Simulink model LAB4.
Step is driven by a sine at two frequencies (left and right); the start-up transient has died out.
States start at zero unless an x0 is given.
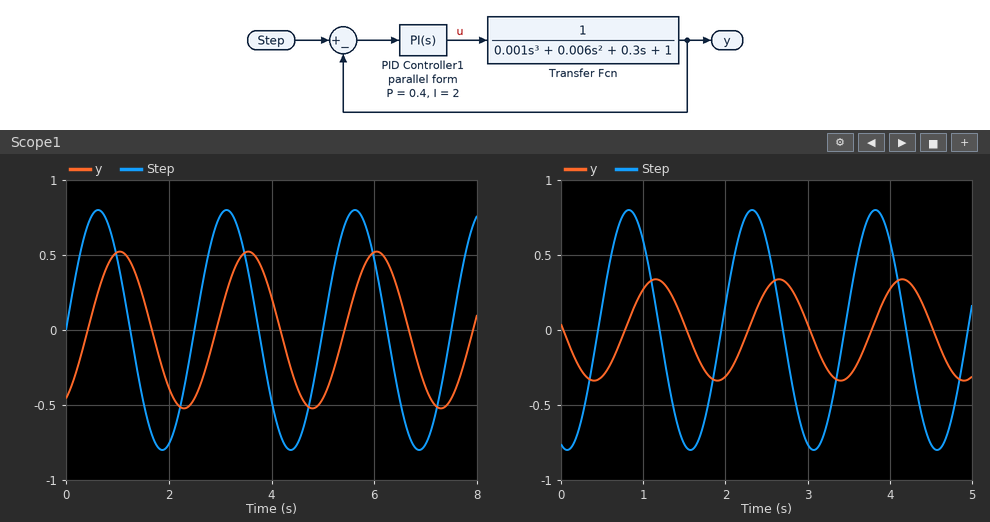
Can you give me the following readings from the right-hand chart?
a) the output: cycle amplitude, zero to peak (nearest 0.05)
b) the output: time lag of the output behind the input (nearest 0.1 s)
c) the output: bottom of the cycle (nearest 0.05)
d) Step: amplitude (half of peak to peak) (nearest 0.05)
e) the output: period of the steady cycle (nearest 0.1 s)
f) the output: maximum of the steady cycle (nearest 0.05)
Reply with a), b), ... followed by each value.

a) 0.35
b) 0.3 s
c) -0.35
d) 0.80
e) 1.5 s
f) 0.35
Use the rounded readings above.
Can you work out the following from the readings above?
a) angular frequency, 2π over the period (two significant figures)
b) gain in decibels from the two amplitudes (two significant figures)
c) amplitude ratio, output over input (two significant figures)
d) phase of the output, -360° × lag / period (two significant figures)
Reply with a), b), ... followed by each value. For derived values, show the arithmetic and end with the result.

a) 2π / 1.5 = 4.2 rad/s
b) 20 log10(0.35 / 0.8) = -7.2 dB
c) 0.35 / 0.8 = 0.44
d) -360 × 0.3 / 1.5 = -72°
